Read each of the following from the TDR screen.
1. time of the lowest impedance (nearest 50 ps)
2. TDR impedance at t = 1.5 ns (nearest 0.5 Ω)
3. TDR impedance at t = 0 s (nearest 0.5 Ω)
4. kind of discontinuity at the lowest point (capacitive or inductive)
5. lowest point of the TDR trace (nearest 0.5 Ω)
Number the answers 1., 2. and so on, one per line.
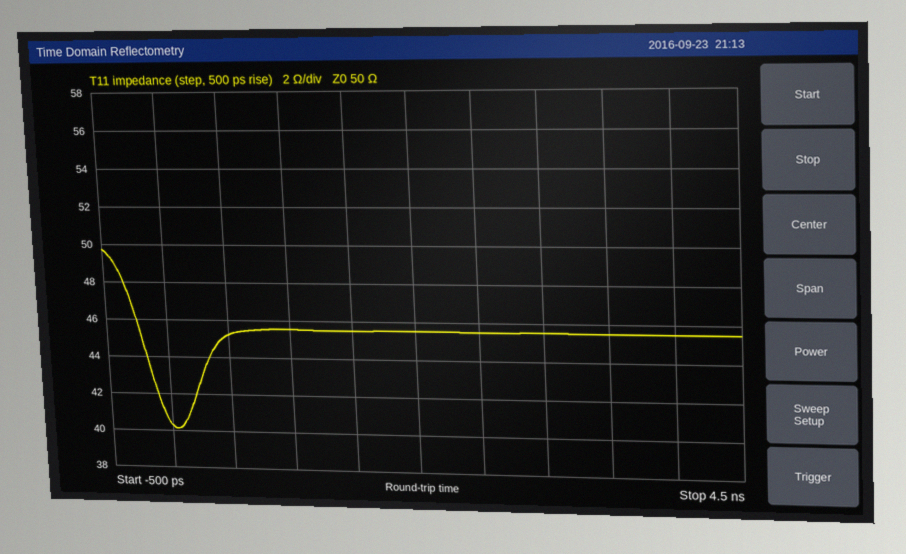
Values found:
1. 50 ps
2. 45.5 Ω
3. 40.5 Ω
4. capacitive
5. 40.0 Ω
